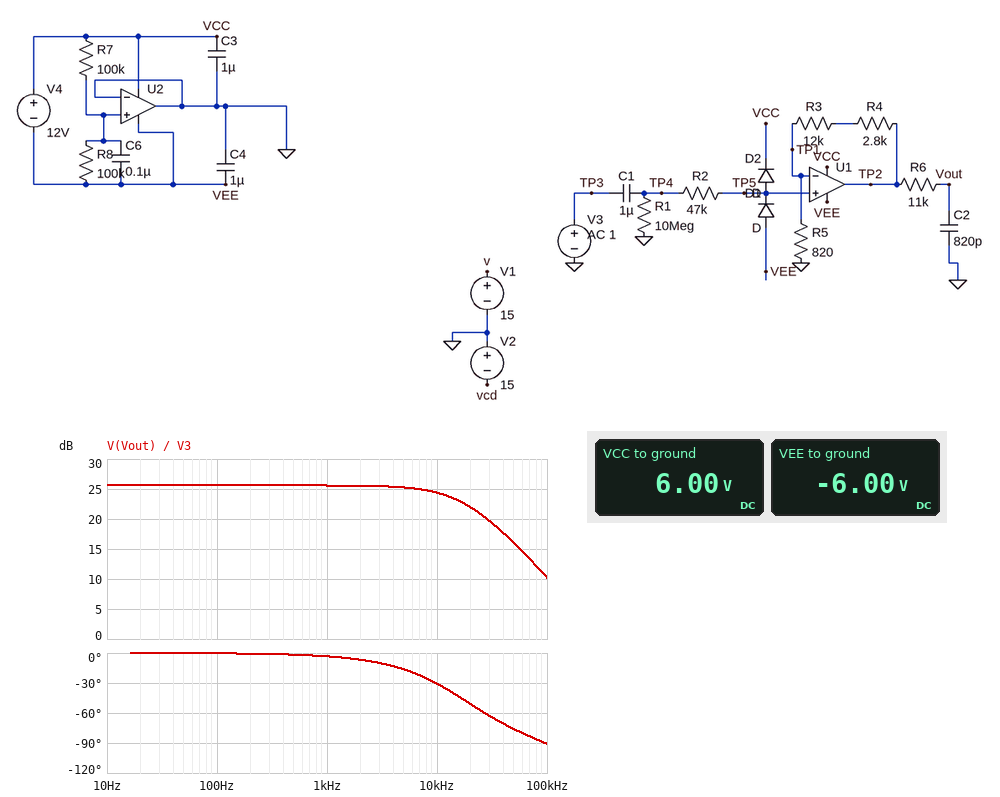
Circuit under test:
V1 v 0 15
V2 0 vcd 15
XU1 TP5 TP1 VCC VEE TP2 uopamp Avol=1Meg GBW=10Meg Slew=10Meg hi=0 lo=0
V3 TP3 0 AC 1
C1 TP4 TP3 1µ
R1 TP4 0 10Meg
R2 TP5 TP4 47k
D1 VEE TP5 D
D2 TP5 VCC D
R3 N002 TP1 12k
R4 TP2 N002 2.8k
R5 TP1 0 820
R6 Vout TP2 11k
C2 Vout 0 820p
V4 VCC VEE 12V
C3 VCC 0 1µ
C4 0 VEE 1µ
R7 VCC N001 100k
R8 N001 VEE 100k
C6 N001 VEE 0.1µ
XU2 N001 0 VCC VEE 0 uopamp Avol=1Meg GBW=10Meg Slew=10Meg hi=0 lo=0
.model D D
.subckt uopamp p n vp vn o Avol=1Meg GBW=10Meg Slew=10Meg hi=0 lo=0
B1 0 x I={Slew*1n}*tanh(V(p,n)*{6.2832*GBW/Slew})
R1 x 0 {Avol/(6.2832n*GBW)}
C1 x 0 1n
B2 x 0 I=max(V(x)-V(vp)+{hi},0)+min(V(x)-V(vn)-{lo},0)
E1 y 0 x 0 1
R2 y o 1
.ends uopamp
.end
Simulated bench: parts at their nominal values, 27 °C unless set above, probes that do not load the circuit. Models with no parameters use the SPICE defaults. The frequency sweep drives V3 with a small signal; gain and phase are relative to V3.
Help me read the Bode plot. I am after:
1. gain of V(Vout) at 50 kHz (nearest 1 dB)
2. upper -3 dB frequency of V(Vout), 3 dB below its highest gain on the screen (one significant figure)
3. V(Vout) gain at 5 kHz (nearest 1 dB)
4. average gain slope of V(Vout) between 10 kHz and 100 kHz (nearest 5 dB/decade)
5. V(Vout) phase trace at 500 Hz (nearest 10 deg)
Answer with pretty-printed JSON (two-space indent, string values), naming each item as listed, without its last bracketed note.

{
  "gain of V(Vout) at 50 kHz": "16 dB",
  "upper -3 dB frequency of V(Vout), 3 dB below its highest gain on the screen": "20 kHz",
  "V(Vout) gain at 5 kHz": "25 dB",
  "average gain slope of V(Vout) between 10 kHz and 100 kHz": "-15 dB/decade",
  "V(Vout) phase trace at 500 Hz": "0 deg"
}
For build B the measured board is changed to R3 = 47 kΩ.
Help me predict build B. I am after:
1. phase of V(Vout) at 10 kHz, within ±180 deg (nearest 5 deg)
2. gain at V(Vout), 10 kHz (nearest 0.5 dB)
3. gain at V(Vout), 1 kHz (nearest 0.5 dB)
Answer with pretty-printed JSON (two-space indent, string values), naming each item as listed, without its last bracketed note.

{
  "phase of V(Vout) at 10 kHz, within ±180 deg": "-35 deg",
  "gain at V(Vout), 10 kHz": "34.5 dB",
  "gain at V(Vout), 1 kHz": "36.0 dB"
}
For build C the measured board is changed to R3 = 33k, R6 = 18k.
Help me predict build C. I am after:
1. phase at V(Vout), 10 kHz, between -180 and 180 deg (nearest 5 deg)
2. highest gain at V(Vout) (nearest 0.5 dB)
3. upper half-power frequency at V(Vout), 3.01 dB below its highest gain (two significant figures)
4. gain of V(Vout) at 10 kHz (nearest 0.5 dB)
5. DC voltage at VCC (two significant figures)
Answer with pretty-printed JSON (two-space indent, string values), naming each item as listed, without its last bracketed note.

{
  "phase at V(Vout), 10 kHz, between -180 and 180 deg": "-45 deg",
  "highest gain at V(Vout)": "33.0 dB",
  "upper half-power frequency at V(Vout), 3.01 dB below its highest gain": "11 kHz",
  "gain of V(Vout) at 10 kHz": "30.5 dB",
  "DC voltage at VCC": "6.0 V"
}
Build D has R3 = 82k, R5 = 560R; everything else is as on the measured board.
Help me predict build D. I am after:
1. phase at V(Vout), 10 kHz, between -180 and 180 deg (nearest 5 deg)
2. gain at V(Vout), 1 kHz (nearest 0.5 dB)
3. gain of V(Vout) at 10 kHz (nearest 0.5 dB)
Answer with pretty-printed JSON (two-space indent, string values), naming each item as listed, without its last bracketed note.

{
  "phase at V(Vout), 10 kHz, between -180 and 180 deg": "-40 deg",
  "gain at V(Vout), 1 kHz": "43.5 dB",
  "gain of V(Vout) at 10 kHz": "42.5 dB"
}
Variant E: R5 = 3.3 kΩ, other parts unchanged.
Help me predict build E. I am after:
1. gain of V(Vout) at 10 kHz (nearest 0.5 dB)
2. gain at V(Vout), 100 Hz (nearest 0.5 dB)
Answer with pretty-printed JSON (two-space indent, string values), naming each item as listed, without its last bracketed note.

{
  "gain of V(Vout) at 10 kHz": "13.5 dB",
  "gain at V(Vout), 100 Hz": "15.0 dB"
}
